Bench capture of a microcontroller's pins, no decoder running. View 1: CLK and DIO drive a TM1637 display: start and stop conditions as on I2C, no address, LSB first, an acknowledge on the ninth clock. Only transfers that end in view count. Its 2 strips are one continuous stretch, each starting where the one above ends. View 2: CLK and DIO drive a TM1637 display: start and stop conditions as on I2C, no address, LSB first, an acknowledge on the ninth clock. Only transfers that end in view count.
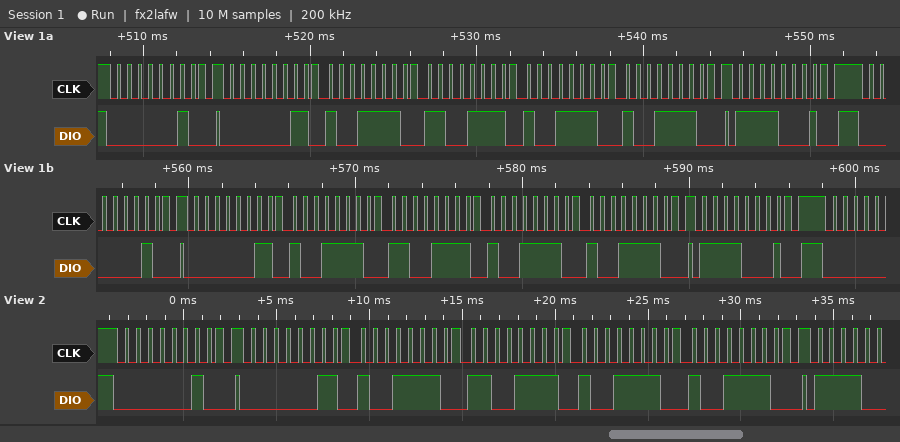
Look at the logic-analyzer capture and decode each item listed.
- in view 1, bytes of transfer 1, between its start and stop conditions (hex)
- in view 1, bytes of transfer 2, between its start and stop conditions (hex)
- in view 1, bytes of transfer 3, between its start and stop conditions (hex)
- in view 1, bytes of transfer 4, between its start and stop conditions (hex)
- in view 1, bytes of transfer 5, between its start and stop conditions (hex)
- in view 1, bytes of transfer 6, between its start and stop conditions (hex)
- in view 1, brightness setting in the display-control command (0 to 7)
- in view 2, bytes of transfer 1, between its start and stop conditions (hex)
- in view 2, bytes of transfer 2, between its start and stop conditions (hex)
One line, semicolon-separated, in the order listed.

40; C0 79 F3 79 79; 8F; 40; C0 79 F3 79 79; 8F; 7; 40; C0 79 F3 79 79
